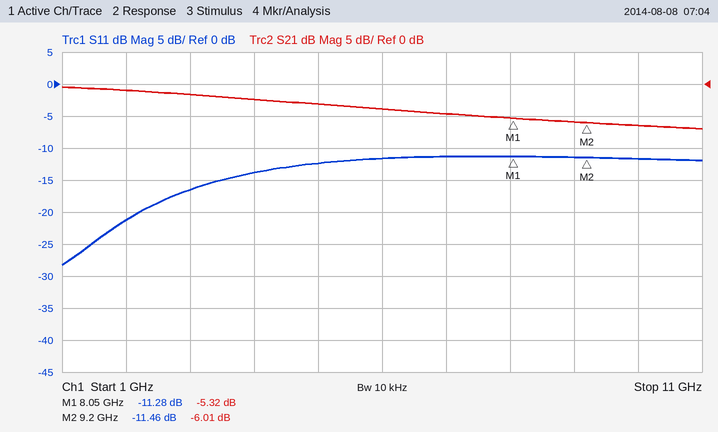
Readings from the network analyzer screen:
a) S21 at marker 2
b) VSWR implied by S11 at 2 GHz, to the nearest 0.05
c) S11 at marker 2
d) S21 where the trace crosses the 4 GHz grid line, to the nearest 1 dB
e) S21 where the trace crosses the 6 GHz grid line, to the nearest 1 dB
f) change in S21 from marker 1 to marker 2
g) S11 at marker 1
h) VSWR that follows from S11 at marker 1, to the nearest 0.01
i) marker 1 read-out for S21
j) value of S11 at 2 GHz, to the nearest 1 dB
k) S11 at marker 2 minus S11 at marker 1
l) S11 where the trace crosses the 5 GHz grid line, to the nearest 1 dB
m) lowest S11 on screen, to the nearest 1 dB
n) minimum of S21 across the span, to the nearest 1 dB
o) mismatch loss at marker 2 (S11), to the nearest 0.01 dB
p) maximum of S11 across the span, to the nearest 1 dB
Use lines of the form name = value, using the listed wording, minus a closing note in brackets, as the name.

S21 at marker 2 = -6.01 dB
VSWR implied by S11 at 2 GHz, to the nearest 0.05 = 1.20
S11 at marker 2 = -11.46 dB
S21 where the trace crosses the 4 GHz grid line, to the nearest 1 dB = -2 dB
S21 where the trace crosses the 6 GHz grid line, to the nearest 1 dB = -4 dB
change in S21 from marker 1 to marker 2 = -0.69 dB
S11 at marker 1 = -11.28 dB
VSWR that follows from S11 at marker 1, to the nearest 0.01 = 1.75
marker 1 read-out for S21 = -5.32 dB
value of S11 at 2 GHz, to the nearest 1 dB = -21 dB
S11 at marker 2 minus S11 at marker 1 = -0.18 dB
S11 where the trace crosses the 5 GHz grid line, to the nearest 1 dB = -12 dB
lowest S11 on screen, to the nearest 1 dB = -28 dB
minimum of S21 across the span, to the nearest 1 dB = -7 dB
mismatch loss at marker 2 (S11), to the nearest 0.01 dB = 0.32 dB
maximum of S11 across the span, to the nearest 1 dB = -11 dB
